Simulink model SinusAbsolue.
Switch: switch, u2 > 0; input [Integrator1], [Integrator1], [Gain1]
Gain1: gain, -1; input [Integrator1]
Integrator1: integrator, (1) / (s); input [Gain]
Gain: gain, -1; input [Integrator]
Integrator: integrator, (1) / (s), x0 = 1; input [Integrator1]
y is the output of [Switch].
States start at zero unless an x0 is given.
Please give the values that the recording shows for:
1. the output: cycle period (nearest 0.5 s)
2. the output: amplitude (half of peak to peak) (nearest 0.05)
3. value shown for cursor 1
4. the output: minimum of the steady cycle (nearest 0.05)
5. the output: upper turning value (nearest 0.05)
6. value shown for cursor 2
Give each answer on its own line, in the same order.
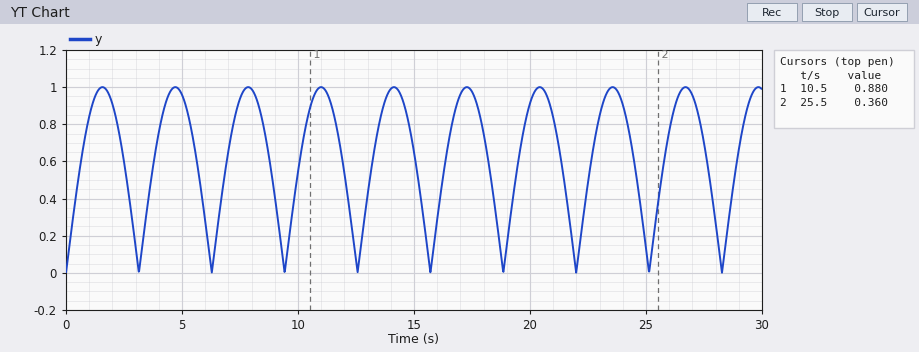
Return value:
3.0 s
0.50
0.880
0.00
1.00
0.360
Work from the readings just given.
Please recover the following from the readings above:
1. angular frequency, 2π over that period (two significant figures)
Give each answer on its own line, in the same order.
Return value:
2.1 rad/s
